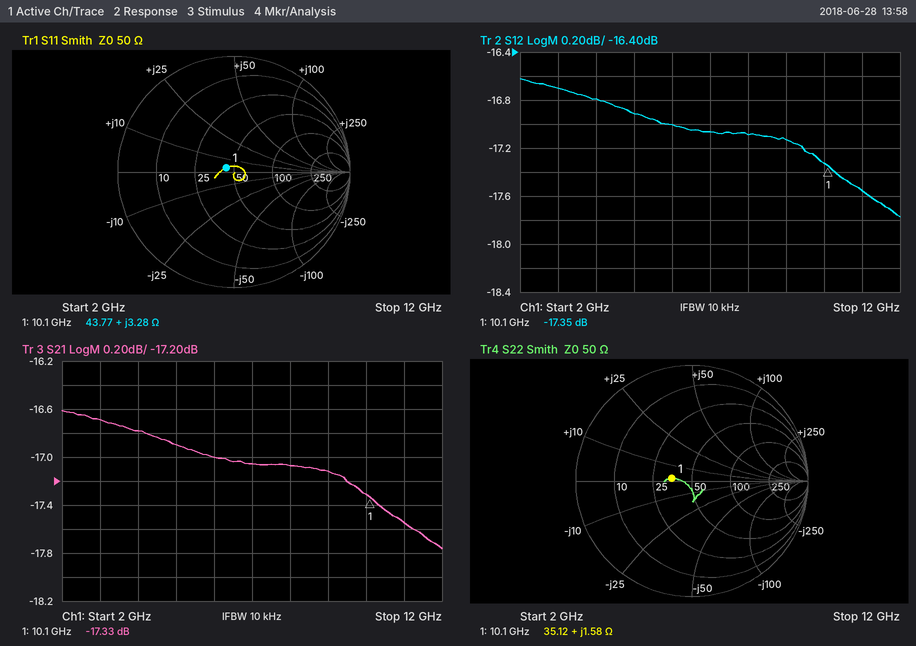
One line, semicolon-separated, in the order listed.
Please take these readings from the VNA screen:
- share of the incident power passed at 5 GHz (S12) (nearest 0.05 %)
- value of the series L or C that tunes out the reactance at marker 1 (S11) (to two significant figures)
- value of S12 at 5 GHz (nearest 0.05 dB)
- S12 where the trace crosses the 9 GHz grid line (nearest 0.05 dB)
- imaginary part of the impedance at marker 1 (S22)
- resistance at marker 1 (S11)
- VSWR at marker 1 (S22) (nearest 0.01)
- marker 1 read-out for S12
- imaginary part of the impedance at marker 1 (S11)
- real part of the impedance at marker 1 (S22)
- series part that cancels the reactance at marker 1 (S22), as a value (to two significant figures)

2.05 %; 4.8 pF; -16.90 dB; -17.15 dB; +1.58 Ω; 43.77 Ω; 1.43; -17.35 dB; +3.28 Ω; 35.12 Ω; 10.0 pF
